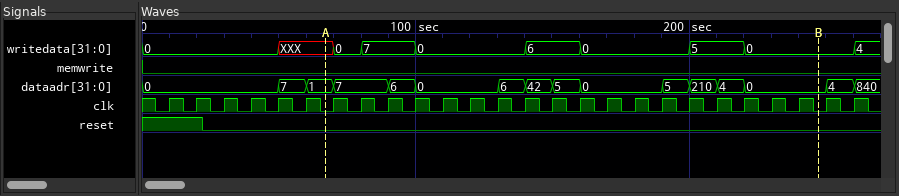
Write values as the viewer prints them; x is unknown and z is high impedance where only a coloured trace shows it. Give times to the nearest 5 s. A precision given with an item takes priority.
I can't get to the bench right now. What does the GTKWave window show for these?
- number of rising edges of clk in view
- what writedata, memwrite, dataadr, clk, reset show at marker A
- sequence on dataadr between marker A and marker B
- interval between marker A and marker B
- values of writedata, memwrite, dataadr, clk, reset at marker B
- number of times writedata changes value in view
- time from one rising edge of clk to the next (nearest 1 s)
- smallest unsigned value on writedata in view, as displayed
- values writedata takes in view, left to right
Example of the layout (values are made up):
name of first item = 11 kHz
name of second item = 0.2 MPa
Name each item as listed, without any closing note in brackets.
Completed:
number of rising edges of clk in view = 26
what writedata, memwrite, dataadr, clk, reset show at marker A = writedata=XXX, memwrite=0, dataadr=1, clk=0, reset=0
sequence on dataadr between marker A and marker B = 1, 7, 6, 0, 6, 42, 5, 0, 5, 210, 4, 0
interval between marker A and marker B = 180 s
values of writedata, memwrite, dataadr, clk, reset at marker B = writedata=0, memwrite=0, dataadr=0, clk=0, reset=0
number of times writedata changes value in view = 9
time from one rising edge of clk to the next = 10 s
smallest unsigned value on writedata in view, as displayed = 0
values writedata takes in view, left to right = 0, XXX, 0, 7, 0, 6, 0, 5, 0, 4
